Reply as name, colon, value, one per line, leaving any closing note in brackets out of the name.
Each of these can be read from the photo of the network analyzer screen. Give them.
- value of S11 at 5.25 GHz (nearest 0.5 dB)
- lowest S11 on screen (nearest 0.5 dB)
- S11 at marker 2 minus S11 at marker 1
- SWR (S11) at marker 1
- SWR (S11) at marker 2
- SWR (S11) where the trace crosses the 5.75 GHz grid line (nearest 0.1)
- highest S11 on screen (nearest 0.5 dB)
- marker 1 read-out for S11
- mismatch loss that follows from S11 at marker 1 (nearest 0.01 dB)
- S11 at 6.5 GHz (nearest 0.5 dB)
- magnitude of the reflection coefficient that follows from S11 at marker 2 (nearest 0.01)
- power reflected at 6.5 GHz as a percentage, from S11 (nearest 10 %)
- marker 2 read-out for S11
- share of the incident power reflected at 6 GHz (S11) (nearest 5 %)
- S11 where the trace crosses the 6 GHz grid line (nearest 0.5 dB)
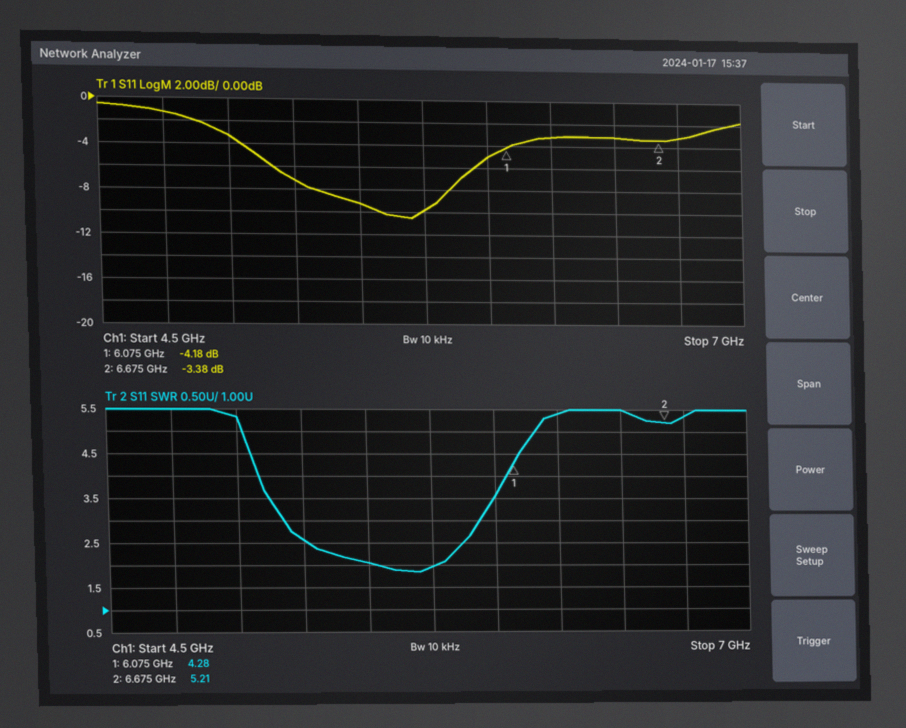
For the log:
value of S11 at 5.25 GHz: -7.0 dB
lowest S11 on screen: -10.5 dB
S11 at marker 2 minus S11 at marker 1: 0.80 dB
SWR (S11) at marker 1: 4.28
SWR (S11) at marker 2: 5.21
SWR (S11) where the trace crosses the 5.75 GHz grid line: 2.0
highest S11 on screen: -0.5 dB
marker 1 read-out for S11: -4.18 dB
mismatch loss that follows from S11 at marker 1: 2.09 dB
S11 at 6.5 GHz: -3.0 dB
magnitude of the reflection coefficient that follows from S11 at marker 2: 0.68
power reflected at 6.5 GHz as a percentage, from S11: 50 %
marker 2 read-out for S11: -3.38 dB
share of the incident power reflected at 6 GHz (S11): 30 %
S11 where the trace crosses the 6 GHz grid line: -5.0 dB
